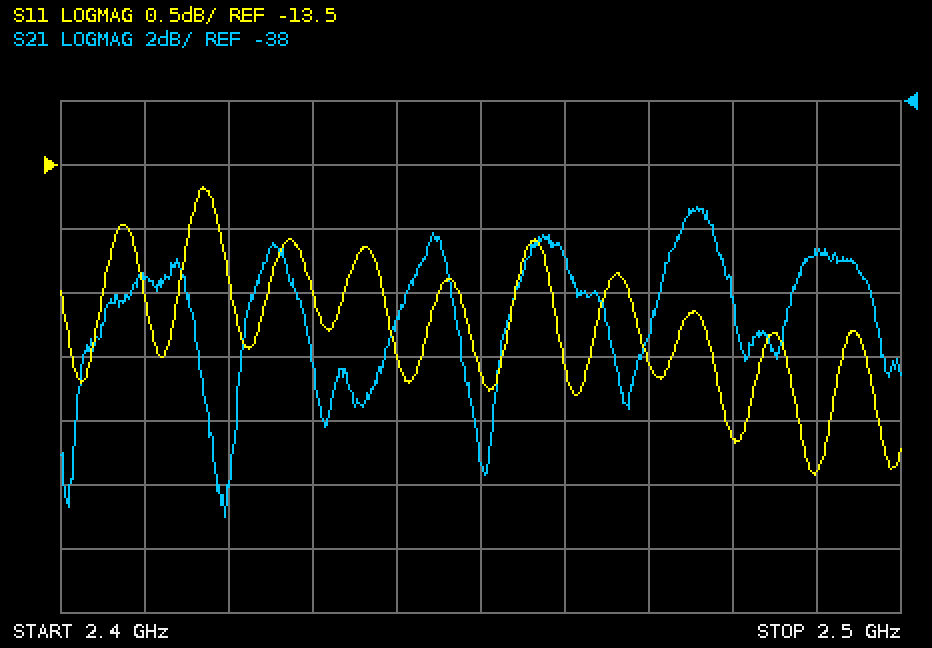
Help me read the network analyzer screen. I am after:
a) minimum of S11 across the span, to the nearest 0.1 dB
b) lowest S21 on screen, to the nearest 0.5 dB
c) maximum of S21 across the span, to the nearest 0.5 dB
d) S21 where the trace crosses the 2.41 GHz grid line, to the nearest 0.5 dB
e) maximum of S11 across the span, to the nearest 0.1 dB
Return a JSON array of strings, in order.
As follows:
["-15.9 dB", "-51.0 dB", "-41.5 dB", "-43.5 dB", "-13.7 dB"]
